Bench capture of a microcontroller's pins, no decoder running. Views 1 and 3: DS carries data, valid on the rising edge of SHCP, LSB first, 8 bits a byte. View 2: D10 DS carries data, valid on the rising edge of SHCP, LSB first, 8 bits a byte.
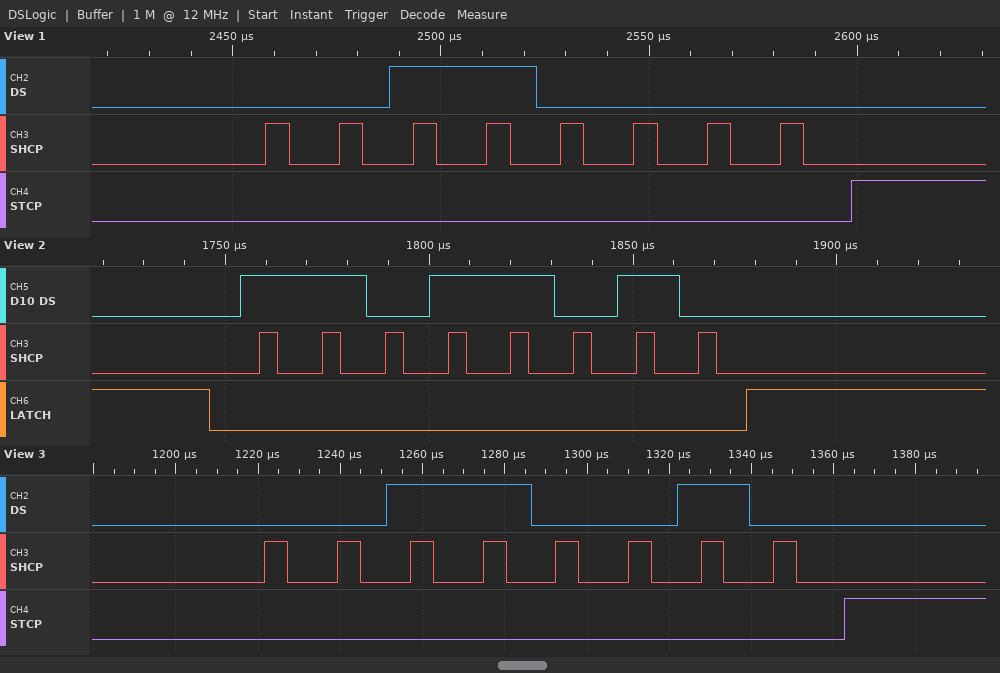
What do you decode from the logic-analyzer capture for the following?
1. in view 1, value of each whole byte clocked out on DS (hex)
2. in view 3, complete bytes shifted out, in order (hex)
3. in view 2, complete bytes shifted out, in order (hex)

0C
4C
0x5B
